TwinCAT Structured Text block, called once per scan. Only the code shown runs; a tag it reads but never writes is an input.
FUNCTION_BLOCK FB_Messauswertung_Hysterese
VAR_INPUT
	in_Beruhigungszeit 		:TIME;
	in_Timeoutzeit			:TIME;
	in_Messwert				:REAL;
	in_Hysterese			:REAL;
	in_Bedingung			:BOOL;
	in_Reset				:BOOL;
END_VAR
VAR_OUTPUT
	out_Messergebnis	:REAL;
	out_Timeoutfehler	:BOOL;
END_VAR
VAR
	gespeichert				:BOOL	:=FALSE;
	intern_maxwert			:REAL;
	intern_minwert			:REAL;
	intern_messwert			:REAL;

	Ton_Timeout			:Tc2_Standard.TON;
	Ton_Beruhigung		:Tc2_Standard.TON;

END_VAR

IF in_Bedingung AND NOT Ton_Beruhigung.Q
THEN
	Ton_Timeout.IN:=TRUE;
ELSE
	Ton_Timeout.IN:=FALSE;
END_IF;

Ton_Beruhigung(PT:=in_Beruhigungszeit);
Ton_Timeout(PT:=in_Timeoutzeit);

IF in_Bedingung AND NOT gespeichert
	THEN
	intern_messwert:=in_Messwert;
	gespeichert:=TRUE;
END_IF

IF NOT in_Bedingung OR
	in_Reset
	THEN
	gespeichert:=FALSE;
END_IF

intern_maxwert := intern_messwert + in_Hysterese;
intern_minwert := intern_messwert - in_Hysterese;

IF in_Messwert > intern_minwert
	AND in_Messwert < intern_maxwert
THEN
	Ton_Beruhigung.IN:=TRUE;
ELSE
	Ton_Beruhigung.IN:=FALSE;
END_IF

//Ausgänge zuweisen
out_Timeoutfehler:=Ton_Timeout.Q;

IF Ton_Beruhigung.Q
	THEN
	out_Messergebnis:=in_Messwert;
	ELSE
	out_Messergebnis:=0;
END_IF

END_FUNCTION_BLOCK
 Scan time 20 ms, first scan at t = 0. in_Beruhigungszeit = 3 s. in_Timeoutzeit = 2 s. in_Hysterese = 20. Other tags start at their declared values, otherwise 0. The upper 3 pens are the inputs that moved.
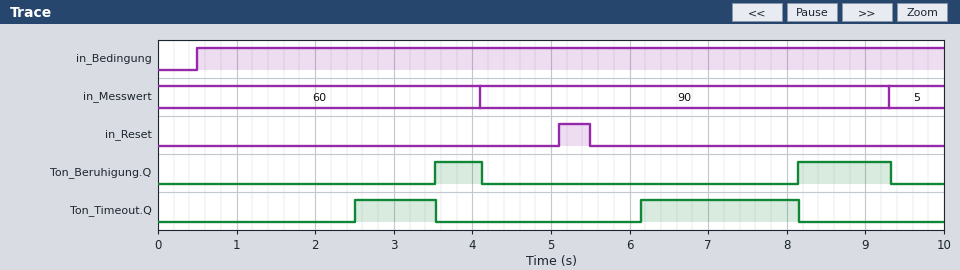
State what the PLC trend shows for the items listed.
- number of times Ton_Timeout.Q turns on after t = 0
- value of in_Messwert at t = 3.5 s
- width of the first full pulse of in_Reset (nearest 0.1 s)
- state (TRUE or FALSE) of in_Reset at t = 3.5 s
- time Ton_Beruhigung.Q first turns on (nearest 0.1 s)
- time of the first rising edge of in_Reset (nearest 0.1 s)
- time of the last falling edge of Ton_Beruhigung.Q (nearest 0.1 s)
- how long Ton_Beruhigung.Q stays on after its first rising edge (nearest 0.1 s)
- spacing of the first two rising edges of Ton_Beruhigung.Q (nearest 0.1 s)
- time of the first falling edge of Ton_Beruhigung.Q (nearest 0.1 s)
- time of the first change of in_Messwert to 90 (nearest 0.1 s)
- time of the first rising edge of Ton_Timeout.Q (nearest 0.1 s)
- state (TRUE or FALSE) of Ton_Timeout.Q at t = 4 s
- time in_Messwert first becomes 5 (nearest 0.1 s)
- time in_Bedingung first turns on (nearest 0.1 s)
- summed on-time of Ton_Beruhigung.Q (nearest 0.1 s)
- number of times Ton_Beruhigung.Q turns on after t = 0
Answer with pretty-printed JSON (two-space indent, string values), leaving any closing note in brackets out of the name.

{
  "number of times Ton_Timeout.Q turns on after t = 0": "2",
  "value of in_Messwert at t = 3.5 s": "60",
  "width of the first full pulse of in_Reset": "0.4 s",
  "state (TRUE or FALSE) of in_Reset at t = 3.5 s": "FALSE",
  "time Ton_Beruhigung.Q first turns on": "3.5 s",
  "time of the first rising edge of in_Reset": "5.1 s",
  "time of the last falling edge of Ton_Beruhigung.Q": "9.3 s",
  "how long Ton_Beruhigung.Q stays on after its first rising edge": "0.6 s",
  "spacing of the first two rising edges of Ton_Beruhigung.Q": "4.6 s",
  "time of the first falling edge of Ton_Beruhigung.Q": "4.1 s",
  "time of the first change of in_Messwert to 90": "4.1 s",
  "time of the first rising edge of Ton_Timeout.Q": "2.5 s",
  "state (TRUE or FALSE) of Ton_Timeout.Q at t = 4 s": "FALSE",
  "time in_Messwert first becomes 5": "9.3 s",
  "time in_Bedingung first turns on": "0.5 s",
  "summed on-time of Ton_Beruhigung.Q": "1.8 s",
  "number of times Ton_Beruhigung.Q turns on after t = 0": "2"
}
